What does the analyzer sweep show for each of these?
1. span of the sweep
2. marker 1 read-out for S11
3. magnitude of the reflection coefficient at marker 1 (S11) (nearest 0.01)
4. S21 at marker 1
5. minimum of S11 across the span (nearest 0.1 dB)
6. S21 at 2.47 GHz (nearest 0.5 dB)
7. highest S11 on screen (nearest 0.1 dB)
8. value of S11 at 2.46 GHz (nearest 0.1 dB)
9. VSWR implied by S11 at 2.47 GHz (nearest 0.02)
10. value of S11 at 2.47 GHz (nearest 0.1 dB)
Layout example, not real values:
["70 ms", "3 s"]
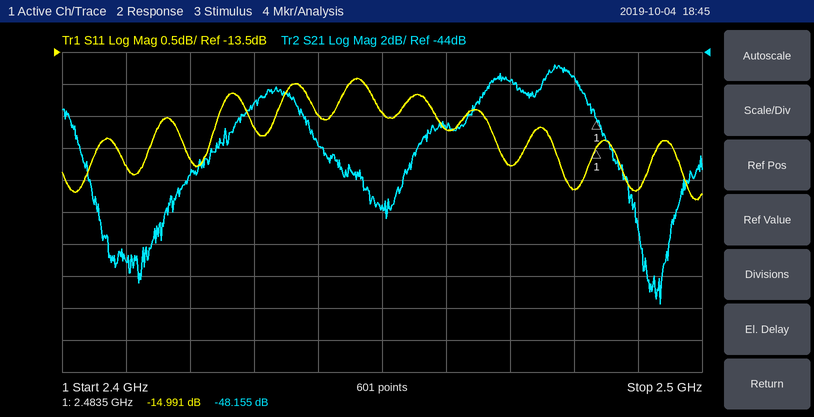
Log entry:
["100 MHz", "-14.991 dB", "0.18", "-48.155 dB", "-15.8 dB", "-46.0 dB", "-13.9 dB", "-14.7 dB", "1.42", "-15.3 dB"]
